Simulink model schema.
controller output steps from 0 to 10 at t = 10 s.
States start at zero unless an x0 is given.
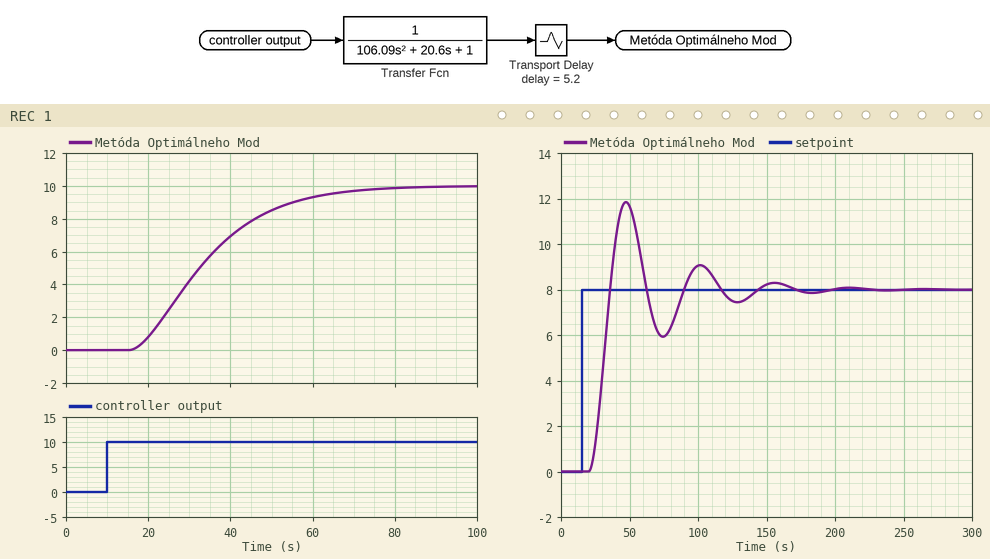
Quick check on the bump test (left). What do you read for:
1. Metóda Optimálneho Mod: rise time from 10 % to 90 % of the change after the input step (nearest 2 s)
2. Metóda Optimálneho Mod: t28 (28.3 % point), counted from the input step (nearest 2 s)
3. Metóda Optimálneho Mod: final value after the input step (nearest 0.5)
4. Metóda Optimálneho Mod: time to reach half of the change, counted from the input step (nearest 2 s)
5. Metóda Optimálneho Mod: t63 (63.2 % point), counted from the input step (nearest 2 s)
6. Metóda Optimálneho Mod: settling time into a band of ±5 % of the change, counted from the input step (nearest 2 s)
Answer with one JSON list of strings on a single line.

["34 s", "16 s", "10.0", "22 s", "28 s", "54 s"]
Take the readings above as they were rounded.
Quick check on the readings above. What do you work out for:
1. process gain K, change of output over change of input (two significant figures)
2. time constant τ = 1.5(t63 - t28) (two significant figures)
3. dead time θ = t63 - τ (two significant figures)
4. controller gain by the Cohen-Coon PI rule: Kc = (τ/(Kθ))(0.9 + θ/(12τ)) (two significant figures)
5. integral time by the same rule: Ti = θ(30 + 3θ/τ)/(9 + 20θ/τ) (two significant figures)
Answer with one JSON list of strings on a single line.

["1.0", "18 s", "10 s", "1.7", "16 s"]
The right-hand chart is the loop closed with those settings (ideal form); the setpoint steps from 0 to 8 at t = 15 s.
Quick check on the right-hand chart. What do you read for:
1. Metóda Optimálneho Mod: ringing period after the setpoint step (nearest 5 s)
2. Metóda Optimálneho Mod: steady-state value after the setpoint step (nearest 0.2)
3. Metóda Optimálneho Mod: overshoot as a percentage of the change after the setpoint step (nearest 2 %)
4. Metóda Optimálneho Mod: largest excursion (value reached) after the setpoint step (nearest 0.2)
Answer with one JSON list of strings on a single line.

["55 s", "8.0", "48 %", "11.8"]
